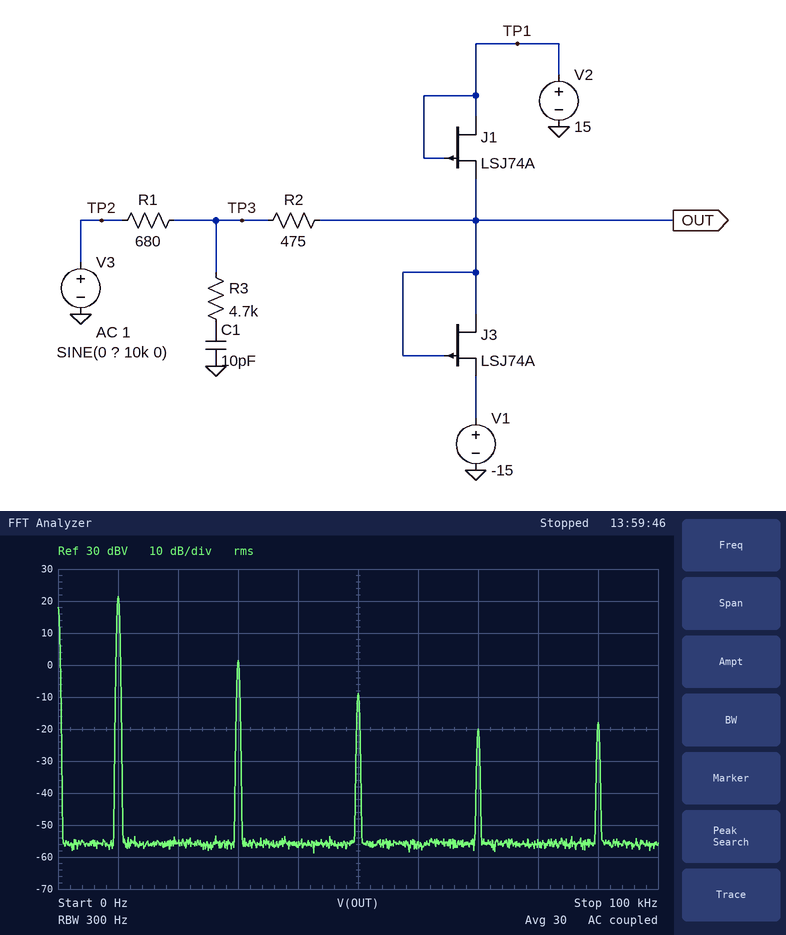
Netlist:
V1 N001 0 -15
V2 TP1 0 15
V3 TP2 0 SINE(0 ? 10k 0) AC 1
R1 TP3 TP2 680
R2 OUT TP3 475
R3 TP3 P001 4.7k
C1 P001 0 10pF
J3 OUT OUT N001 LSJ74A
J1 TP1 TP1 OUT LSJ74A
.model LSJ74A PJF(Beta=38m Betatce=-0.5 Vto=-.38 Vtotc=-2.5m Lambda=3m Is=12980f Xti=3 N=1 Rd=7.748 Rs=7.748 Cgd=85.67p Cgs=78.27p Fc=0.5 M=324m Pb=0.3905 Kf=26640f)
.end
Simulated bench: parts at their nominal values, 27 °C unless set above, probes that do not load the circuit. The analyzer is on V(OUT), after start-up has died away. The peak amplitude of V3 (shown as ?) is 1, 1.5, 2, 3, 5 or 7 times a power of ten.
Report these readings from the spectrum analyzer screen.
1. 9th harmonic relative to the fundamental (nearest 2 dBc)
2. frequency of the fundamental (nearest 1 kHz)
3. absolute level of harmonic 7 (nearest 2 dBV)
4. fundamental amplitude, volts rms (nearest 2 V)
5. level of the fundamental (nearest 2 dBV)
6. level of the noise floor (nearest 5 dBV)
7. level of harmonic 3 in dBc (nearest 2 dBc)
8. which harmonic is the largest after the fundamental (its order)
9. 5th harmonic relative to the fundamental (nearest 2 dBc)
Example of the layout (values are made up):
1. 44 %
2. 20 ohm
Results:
1. -40 dBc
2. 10 kHz
3. -20 dBV
4. 12 V
5. 22 dBV
6. -55 dBV
7. -20 dBc
8. 3
9. -30 dBc
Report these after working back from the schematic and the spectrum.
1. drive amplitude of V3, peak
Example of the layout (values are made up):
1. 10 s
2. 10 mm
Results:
1. 20 V
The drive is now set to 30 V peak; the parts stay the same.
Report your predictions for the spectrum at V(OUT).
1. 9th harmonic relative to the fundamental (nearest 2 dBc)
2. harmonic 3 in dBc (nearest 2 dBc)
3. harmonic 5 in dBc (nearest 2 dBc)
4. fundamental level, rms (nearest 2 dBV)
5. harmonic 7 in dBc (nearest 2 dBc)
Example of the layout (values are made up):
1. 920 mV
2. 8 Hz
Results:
1. -34 dBc
2. -14 dBc
3. -28 dBc
4. 22 dBV
5. -36 dBc
